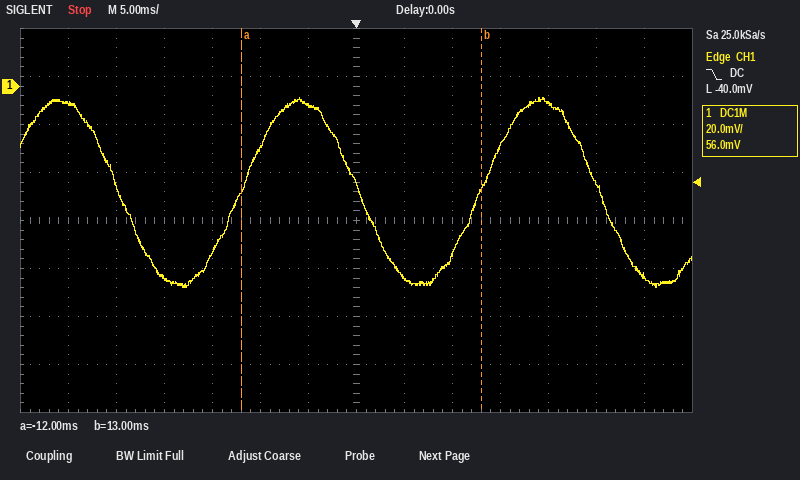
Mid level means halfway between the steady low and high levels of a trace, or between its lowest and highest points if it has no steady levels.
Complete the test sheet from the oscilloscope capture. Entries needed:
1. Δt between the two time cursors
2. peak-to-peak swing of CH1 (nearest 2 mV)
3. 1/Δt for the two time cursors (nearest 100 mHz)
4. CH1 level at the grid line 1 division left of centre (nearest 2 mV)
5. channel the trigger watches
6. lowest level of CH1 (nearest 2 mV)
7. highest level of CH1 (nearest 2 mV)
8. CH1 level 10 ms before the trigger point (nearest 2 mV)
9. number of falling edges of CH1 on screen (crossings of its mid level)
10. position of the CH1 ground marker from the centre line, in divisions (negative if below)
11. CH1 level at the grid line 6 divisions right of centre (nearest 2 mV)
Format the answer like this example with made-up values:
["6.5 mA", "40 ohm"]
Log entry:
["25.0 ms", "80 mV", "40.0 Hz", "-8 mV", "CH1", "-84 mV", "-4 mV", "-26 mV", "3", "+2.8 div", "-80 mV"]
